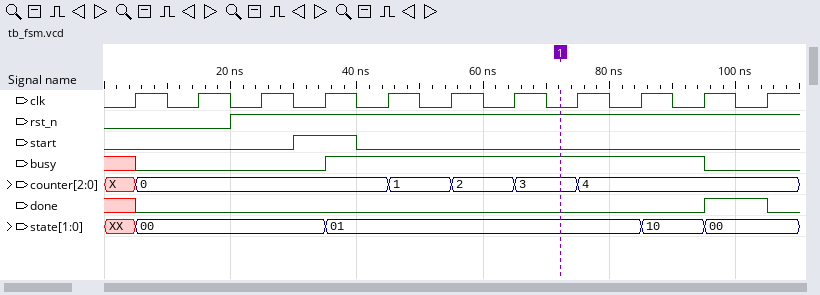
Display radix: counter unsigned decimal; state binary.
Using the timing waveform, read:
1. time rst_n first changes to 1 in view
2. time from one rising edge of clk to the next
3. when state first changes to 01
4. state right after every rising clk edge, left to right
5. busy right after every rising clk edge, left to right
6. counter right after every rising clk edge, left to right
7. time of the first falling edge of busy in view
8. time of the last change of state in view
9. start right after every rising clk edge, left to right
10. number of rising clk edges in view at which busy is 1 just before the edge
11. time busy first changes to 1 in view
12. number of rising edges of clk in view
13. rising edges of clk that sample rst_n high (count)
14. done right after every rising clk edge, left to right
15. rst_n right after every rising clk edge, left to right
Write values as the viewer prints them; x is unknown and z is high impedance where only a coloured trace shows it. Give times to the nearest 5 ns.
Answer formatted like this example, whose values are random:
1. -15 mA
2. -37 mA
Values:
1. 20 ns
2. 10 ns
3. 35 ns
4. 00, 00, 00, 01, 01, 01, 01, 01, 10, 00, 00
5. 0 0 0 1 1 1 1 1 1 0 0
6. 0, 0, 0, 0, 1, 2, 3, 4, 4, 4, 4
7. 95 ns
8. 95 ns
9. 0 0 0 1 0 0 0 0 0 0 0
10. 6
11. 35 ns
12. 11
13. 9
14. 0 0 0 0 0 0 0 0 0 1 0
15. 0 0 1 1 1 1 1 1 1 1 1
